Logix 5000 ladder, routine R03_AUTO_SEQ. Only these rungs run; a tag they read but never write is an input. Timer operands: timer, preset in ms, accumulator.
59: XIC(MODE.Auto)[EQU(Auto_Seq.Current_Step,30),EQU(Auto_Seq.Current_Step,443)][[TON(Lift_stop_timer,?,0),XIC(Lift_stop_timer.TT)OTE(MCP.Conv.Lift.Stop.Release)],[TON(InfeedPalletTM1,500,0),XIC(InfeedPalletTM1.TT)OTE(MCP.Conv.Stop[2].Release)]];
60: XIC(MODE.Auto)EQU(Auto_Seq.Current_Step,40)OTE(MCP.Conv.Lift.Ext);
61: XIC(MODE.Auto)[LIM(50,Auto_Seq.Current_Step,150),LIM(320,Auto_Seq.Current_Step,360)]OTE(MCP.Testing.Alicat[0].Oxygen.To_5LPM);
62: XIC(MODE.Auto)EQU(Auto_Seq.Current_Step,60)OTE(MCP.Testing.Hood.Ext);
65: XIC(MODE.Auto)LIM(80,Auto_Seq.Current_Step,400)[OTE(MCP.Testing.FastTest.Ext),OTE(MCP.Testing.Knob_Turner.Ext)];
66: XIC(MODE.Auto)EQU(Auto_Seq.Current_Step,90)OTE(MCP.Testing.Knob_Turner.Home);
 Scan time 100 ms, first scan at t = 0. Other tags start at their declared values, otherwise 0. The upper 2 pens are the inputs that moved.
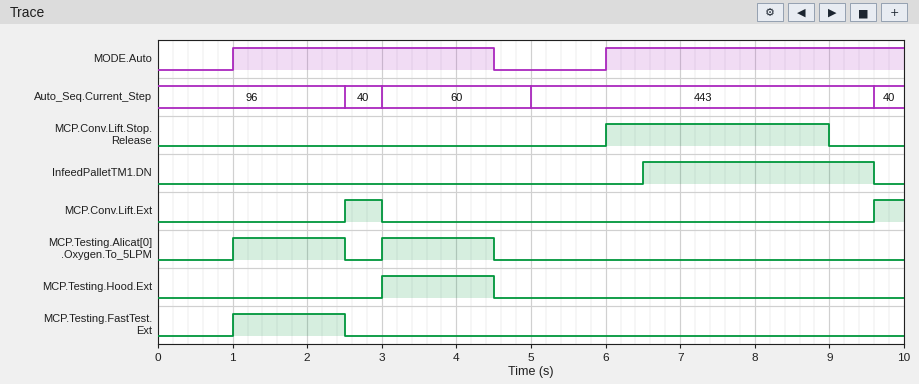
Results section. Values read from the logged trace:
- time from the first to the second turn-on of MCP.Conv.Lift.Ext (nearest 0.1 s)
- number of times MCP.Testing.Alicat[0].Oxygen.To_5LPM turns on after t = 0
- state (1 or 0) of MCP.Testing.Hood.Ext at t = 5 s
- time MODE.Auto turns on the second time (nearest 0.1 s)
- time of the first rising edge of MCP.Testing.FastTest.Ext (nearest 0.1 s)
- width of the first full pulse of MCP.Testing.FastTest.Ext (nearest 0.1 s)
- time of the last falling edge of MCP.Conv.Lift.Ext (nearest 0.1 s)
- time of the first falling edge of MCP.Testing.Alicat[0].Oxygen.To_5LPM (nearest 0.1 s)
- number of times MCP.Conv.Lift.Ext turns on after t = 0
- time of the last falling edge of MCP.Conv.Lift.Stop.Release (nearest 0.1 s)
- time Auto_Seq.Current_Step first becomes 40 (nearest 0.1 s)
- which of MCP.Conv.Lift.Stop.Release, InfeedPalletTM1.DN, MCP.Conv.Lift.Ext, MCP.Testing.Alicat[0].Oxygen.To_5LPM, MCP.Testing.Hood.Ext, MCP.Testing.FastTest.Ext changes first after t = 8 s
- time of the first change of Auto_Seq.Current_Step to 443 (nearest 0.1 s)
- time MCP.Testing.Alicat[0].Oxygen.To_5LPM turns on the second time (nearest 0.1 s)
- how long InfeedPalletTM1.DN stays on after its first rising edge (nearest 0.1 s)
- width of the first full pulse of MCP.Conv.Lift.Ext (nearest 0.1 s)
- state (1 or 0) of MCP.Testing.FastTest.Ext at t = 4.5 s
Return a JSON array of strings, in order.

["7.1 s", "2", "0", "6.0 s", "1.0 s", "1.5 s", "3.0 s", "2.5 s", "2", "9.0 s", "2.5 s", "MCP.Conv.Lift.Stop.Release", "5.0 s", "3.0 s", "3.1 s", "0.5 s", "0"]
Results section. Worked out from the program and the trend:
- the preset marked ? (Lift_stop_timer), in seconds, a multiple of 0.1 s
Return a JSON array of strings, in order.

["3.0 s"]
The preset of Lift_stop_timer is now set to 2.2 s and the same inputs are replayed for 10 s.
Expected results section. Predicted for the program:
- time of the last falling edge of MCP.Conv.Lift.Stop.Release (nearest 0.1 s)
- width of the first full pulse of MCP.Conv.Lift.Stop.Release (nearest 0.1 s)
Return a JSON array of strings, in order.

["8.2 s", "2.2 s"]
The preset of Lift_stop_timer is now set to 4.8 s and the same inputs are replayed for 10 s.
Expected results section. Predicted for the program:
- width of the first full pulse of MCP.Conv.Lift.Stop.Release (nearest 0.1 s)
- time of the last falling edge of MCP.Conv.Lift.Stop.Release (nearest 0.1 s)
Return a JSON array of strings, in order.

["3.6 s", "9.6 s"]
